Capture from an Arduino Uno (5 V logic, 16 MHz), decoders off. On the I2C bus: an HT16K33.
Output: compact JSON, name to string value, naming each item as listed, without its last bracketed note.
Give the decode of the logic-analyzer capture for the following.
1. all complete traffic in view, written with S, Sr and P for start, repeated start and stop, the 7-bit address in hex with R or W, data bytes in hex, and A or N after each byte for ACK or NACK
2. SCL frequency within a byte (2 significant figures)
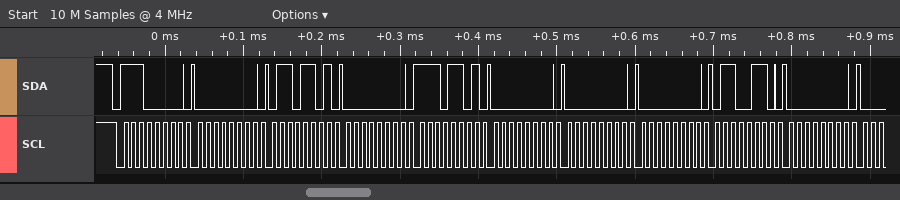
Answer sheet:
{"all complete traffic in view, written with S, Sr and P for start, repeated start and stop, the 7-bit address in hex with R or W, data bytes in hex, and A or N after each byte for ACK or NACK": "S 70W A 00 A 6D A 00 A ED A 00 A 00 A 00 A 66 A 00 A", "SCL frequency within a byte": "100 kHz"}
